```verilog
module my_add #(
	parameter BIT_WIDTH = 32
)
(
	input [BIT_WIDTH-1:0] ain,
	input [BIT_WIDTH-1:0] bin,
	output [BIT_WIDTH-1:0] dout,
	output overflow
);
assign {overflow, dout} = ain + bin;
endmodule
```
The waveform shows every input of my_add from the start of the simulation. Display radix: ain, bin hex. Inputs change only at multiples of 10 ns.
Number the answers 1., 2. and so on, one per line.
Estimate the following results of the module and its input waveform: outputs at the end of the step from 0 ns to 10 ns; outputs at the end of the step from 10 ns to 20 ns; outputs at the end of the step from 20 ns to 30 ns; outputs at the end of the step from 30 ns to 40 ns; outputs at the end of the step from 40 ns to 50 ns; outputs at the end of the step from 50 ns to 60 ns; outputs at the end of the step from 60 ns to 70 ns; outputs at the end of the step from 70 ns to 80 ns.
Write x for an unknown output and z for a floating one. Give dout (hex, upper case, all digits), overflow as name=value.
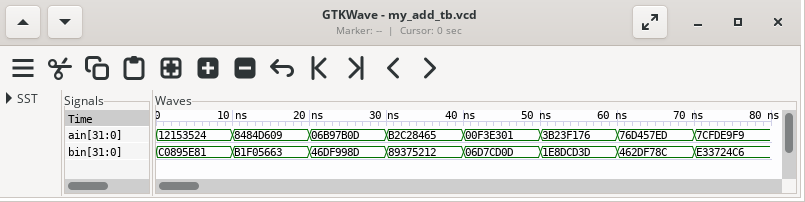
1. dout=D29E93A5, overflow=0
2. dout=36752C6C, overflow=1
3. dout=4D99149A, overflow=0
4. dout=3BF9D677, overflow=1
5. dout=07CBB00E, overflow=0
6. dout=59B1BEB3, overflow=0
7. dout=BD024F79, overflow=0
8. dout=60350EBF, overflow=1
